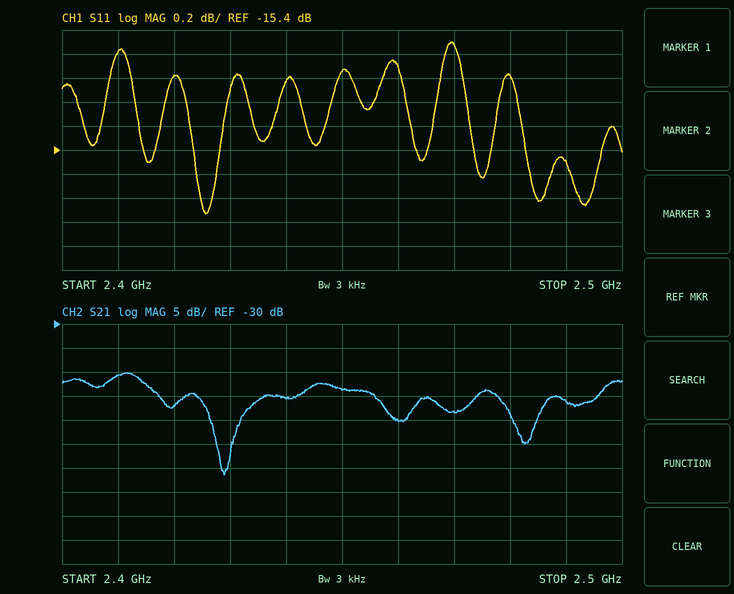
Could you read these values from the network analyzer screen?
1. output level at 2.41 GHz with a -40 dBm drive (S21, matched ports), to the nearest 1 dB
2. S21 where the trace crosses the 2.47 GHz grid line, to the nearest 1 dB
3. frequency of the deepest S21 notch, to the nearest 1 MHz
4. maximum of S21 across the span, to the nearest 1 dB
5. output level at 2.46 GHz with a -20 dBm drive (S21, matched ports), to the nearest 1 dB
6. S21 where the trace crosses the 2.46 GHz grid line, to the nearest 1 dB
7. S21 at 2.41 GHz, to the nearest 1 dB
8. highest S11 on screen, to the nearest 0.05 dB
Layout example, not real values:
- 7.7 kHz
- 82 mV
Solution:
- -81 dBm
- -48 dB
- 2.429 GHz
- -40 dB
- -70 dBm
- -50 dB
- -41 dB
- -14.50 dB
